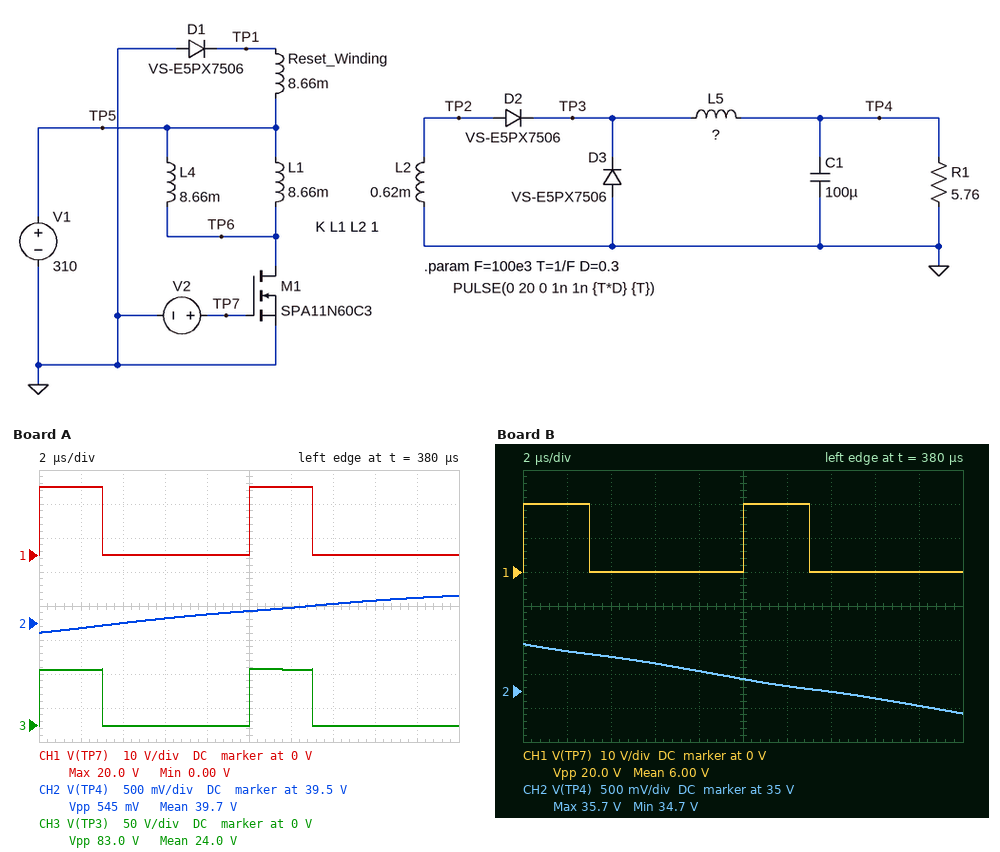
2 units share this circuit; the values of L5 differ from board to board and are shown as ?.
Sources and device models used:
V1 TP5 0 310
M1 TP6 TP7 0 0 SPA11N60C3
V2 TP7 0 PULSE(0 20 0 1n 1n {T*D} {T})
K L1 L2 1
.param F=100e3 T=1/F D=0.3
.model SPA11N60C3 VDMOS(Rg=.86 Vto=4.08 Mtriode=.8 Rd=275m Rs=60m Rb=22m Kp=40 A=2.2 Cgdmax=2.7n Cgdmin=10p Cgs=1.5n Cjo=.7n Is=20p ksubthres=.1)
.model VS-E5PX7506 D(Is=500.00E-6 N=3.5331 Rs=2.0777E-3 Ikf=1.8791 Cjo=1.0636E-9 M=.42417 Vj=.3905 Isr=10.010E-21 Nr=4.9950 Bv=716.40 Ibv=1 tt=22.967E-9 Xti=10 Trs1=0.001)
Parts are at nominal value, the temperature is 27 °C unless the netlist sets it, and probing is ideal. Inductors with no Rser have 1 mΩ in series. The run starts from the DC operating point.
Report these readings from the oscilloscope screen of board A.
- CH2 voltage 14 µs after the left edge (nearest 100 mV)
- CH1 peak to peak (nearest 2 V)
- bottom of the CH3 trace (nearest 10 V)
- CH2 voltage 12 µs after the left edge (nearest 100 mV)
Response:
39.8 V
20 V
0 V
39.7 V
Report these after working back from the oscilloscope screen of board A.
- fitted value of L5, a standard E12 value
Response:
180 µH
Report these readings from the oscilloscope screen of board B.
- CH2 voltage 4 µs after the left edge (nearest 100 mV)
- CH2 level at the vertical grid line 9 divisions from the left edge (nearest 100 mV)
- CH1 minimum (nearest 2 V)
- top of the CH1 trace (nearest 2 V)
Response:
35.5 V
34.8 V
0 V
20 V
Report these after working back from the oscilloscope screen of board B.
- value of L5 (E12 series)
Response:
68 µH
